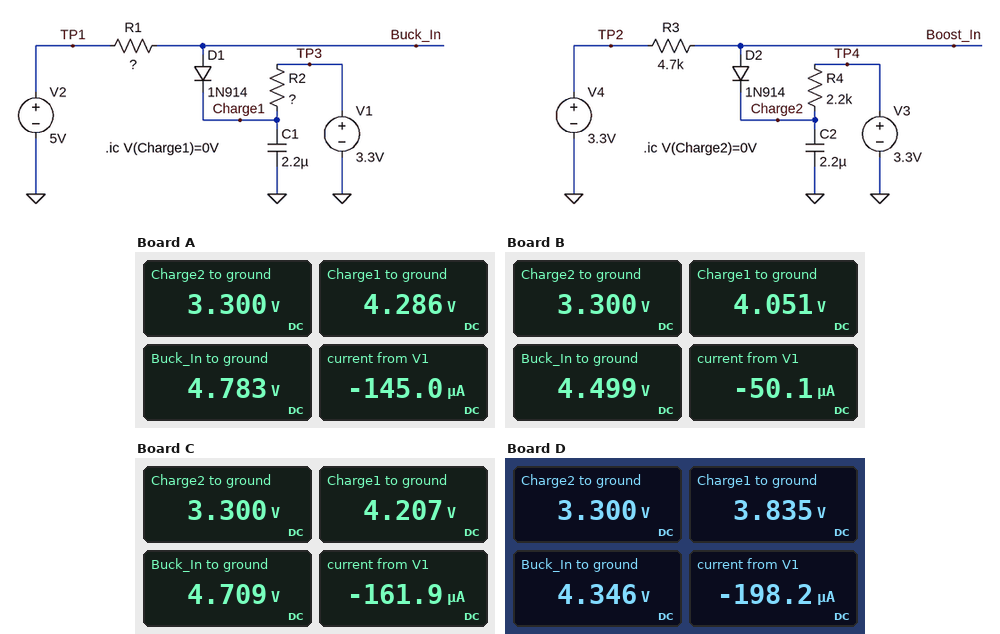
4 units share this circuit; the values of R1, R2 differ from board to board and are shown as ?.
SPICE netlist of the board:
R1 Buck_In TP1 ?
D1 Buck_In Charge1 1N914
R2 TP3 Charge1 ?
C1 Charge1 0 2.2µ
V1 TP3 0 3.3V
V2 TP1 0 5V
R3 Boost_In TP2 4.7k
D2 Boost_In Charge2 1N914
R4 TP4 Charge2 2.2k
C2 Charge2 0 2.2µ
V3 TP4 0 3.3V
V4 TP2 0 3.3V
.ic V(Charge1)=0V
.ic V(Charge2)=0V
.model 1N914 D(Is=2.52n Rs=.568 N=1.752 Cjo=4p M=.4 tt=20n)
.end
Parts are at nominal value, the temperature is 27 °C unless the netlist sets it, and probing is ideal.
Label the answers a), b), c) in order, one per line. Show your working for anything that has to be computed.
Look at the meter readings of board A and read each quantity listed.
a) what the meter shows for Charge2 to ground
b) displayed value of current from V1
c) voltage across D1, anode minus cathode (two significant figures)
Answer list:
a) 3.300 V
b) -145.0 µA
c) 4.783 V - 4.286 V = 500 mV
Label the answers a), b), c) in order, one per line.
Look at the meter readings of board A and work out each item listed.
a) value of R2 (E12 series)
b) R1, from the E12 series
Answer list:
a) 6.8 kΩ
b) 1.5 kΩ
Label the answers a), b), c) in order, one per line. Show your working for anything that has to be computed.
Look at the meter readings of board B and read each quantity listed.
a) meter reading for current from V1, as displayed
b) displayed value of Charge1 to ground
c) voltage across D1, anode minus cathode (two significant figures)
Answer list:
a) -50.1 µA
b) 4.051 V
c) 4.499 V - 4.051 V = 450 mV
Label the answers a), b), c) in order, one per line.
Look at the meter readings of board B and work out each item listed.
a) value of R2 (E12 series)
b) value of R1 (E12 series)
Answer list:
a) 15 kΩ
b) 10 kΩ
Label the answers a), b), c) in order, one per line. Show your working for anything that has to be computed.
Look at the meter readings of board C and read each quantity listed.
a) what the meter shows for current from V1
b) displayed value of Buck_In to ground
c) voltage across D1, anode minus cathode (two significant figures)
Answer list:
a) -161.9 µA
b) 4.709 V
c) 4.709 V - 4.207 V = 500 mV
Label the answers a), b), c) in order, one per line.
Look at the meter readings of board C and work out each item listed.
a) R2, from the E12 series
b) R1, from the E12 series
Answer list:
a) 5.6 kΩ
b) 1.8 kΩ
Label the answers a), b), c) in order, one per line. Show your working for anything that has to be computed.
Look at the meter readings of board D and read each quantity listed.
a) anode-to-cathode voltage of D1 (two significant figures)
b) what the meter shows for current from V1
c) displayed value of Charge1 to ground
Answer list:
a) 4.346 V - 3.835 V = 510 mV
b) -198.2 µA
c) 3.835 V
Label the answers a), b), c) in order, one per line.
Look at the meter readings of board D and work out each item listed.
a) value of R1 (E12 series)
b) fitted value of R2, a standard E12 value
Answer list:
a) 3.3 kΩ
b) 2.7 kΩ
